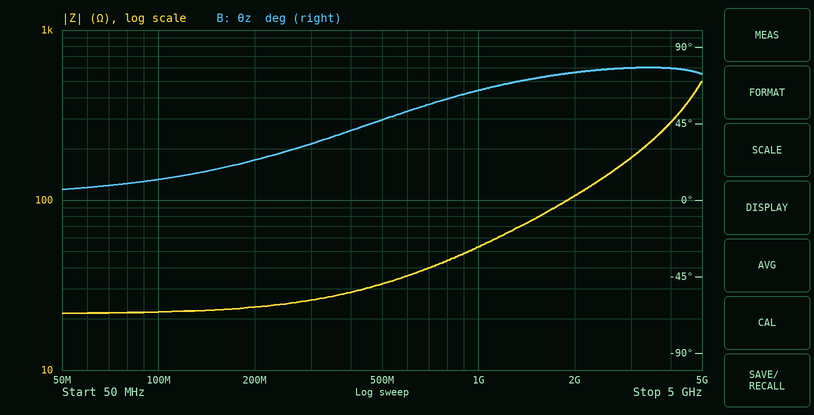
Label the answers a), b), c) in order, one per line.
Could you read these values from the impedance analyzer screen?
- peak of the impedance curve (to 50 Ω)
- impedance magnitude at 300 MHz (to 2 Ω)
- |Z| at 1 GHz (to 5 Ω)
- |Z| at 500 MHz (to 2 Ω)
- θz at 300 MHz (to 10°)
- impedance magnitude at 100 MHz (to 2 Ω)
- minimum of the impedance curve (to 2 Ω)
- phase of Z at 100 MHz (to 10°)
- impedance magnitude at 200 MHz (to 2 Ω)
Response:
a) 500 Ω
b) 26 Ω
c) 55 Ω
d) 32 Ω
e) 30°
f) 22 Ω
g) 22 Ω
h) 10°
i) 24 Ω
